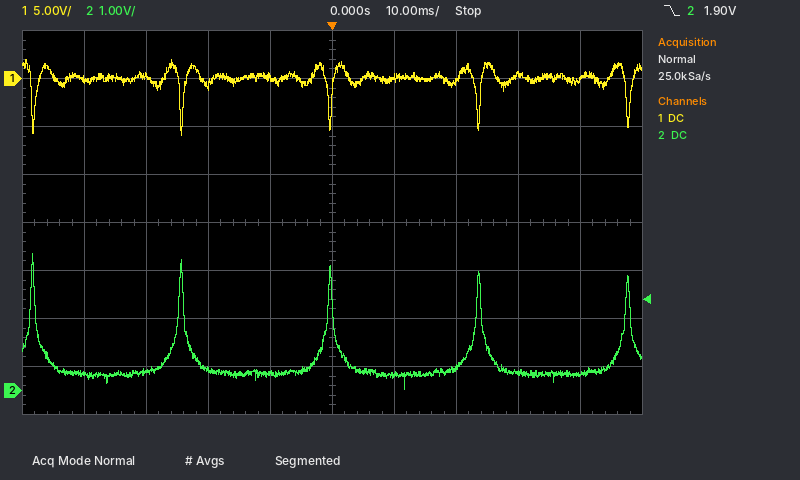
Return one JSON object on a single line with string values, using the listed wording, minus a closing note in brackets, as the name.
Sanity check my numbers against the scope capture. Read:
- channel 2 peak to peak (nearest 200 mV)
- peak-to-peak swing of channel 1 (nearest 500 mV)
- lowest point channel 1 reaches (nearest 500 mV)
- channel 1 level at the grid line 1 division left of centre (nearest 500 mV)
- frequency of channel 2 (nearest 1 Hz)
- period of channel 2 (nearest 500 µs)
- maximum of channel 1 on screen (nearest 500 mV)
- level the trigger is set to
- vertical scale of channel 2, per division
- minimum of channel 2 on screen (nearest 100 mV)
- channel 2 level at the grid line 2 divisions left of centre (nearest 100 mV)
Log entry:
{"channel 2 peak to peak": "2.8 V", "peak-to-peak swing of channel 1": "8.0 V", "lowest point channel 1 reaches": "-6.0 V", "channel 1 level at the grid line 1 division left of centre": "0.0 V", "frequency of channel 2": "42 Hz", "period of channel 2": "24.0 ms", "maximum of channel 1 on screen": "2.0 V", "level the trigger is set to": "1.90 V", "vertical scale of channel 2, per division": "1 V", "minimum of channel 2 on screen": "0.0 V", "channel 2 level at the grid line 2 divisions left of centre": "400 mV"}
